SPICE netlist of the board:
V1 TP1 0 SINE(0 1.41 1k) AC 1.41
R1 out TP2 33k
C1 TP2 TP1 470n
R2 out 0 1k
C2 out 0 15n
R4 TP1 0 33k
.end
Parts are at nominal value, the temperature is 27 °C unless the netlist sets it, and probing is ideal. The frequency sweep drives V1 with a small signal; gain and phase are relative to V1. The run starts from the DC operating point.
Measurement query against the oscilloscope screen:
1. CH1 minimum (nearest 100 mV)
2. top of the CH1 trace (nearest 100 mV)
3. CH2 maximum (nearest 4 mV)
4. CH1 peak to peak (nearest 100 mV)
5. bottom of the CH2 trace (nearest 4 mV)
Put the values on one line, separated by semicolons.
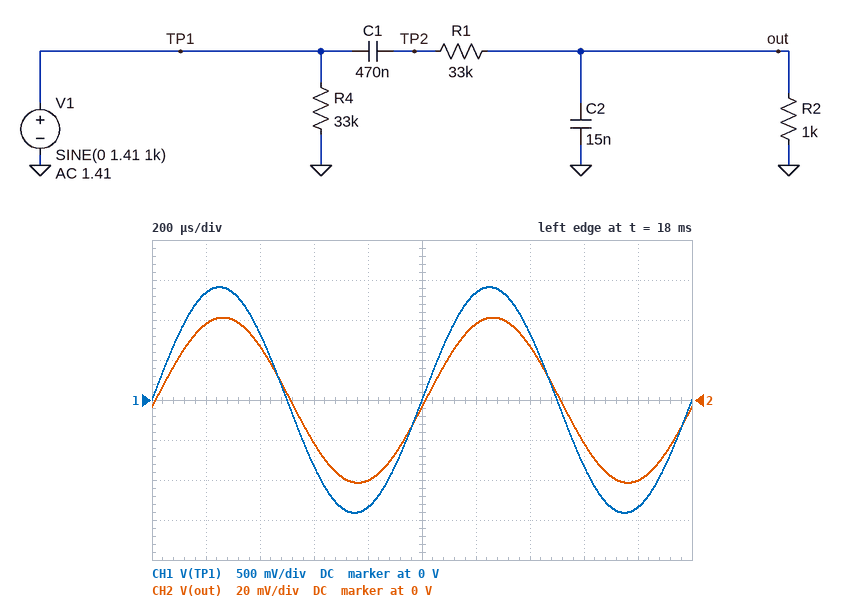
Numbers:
-1.4 V; 1.4 V; 40 mV; 2.8 V; -40 mV
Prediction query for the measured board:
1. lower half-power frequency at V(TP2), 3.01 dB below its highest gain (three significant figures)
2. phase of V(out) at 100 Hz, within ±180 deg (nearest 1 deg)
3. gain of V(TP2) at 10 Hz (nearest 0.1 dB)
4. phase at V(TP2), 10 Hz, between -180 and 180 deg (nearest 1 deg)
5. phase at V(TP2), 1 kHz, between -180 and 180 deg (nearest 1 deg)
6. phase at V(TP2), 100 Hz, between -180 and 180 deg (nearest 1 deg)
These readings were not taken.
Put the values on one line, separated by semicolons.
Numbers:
9.96 Hz; 5 deg; -3.0 dB; 45 deg; 1 deg; 6 deg
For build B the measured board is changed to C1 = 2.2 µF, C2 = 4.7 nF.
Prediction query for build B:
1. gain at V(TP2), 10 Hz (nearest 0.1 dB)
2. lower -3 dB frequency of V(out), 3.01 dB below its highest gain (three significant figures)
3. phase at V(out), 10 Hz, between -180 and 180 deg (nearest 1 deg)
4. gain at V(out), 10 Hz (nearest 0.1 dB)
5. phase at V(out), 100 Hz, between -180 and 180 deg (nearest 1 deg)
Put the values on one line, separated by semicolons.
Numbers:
-0.2 dB; 2.13 Hz; 12 deg; -30.8 dB; 1 deg
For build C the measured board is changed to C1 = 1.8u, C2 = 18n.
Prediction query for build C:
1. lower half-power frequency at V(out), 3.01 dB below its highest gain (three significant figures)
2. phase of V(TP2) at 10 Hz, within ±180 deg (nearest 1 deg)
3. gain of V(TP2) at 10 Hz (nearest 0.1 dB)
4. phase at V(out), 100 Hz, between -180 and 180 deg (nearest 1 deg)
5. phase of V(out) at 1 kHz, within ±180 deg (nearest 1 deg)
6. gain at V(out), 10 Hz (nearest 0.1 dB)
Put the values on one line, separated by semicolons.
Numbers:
2.60 Hz; 15 deg; -0.3 dB; 1 deg; -6 deg; -30.9 dB
